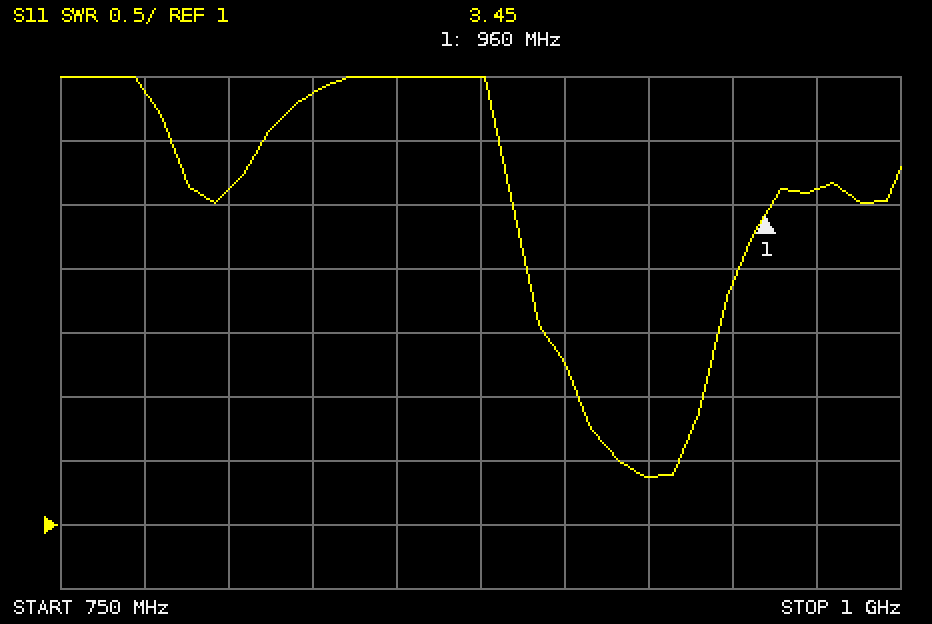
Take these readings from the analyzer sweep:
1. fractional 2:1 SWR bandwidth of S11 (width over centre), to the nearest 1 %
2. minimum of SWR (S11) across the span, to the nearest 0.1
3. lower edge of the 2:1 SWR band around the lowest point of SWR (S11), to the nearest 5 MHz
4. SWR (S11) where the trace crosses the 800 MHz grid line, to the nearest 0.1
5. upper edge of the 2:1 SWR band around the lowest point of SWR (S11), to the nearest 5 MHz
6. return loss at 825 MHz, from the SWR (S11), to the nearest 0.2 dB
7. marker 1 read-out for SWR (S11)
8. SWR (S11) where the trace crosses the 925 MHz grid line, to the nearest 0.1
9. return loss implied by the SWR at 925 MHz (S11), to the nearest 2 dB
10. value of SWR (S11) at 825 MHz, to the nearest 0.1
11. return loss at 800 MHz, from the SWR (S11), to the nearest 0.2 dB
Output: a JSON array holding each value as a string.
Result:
["4 %", "1.4", "905 MHz", "3.6", "940 MHz", "4.0 dB", "3.45", "1.4", "16 dB", "4.4", "5.0 dB"]
